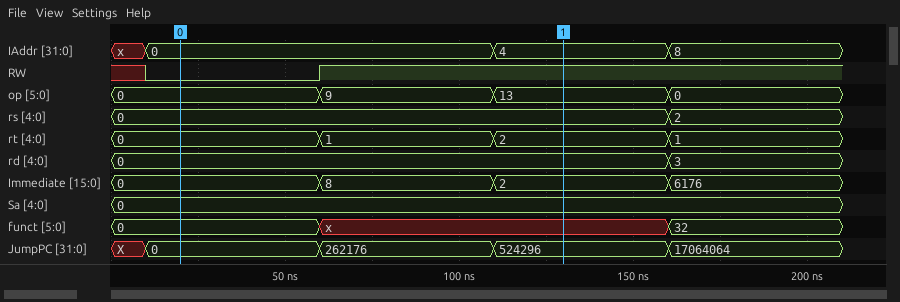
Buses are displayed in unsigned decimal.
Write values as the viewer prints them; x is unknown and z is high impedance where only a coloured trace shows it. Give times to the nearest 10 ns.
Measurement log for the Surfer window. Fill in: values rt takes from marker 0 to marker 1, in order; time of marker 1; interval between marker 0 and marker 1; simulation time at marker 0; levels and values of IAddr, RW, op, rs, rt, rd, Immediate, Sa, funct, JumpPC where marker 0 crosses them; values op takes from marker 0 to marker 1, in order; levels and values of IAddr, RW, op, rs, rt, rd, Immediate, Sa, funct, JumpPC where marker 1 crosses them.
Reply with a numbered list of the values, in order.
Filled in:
1. 0, 1, 2
2. 130 ns
3. 110 ns
4. 20 ns
5. IAddr=0, RW=0, op=0, rs=0, rt=0, rd=0, Immediate=0, Sa=0, funct=0, JumpPC=0
6. 0, 9, 13
7. IAddr=4, RW=1, op=13, rs=0, rt=2, rd=0, Immediate=2, Sa=0, funct=x, JumpPC=524296
